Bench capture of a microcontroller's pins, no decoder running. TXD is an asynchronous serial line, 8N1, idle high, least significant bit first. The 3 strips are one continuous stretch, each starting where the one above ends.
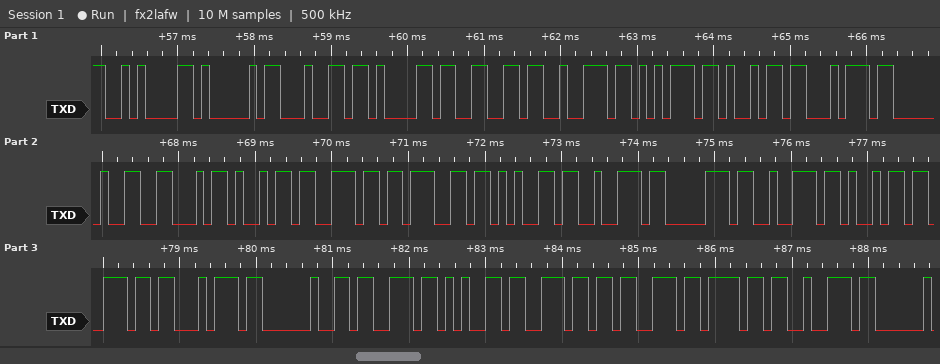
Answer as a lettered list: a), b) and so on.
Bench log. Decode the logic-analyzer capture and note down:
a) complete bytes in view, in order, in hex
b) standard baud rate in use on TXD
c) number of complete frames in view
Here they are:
a) 0A 41 64 61 66 72 75 69 74 20 46 69 6E 67 65 72 70 72 69 6E 74 20 73 65 6E 73 6F 72
b) 9600 baud
c) 28
